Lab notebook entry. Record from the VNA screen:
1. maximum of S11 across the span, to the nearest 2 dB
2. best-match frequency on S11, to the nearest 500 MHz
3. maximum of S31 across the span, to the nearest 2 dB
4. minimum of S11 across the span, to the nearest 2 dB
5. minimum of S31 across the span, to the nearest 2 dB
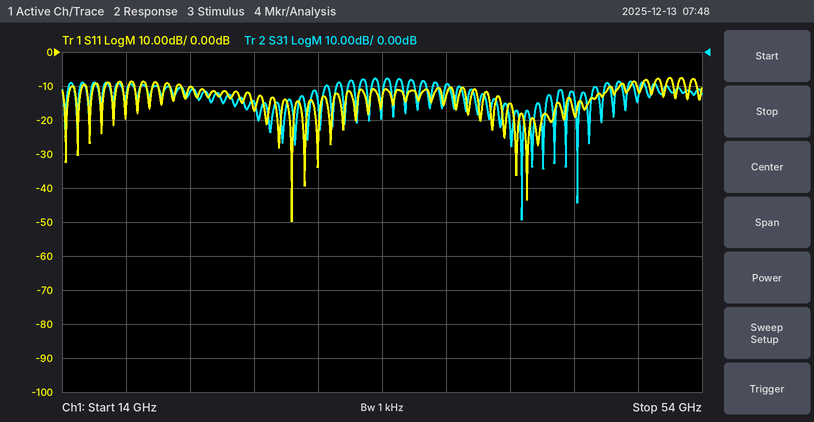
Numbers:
-8 dB
28.5 GHz
-8 dB
-50 dB
-50 dB
